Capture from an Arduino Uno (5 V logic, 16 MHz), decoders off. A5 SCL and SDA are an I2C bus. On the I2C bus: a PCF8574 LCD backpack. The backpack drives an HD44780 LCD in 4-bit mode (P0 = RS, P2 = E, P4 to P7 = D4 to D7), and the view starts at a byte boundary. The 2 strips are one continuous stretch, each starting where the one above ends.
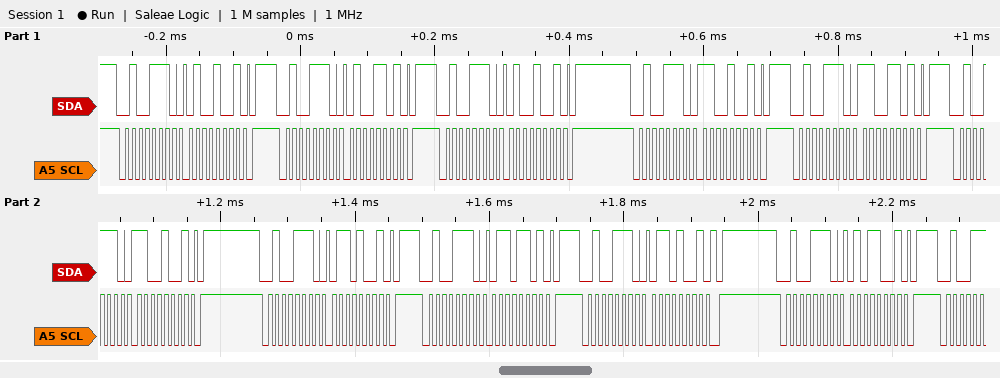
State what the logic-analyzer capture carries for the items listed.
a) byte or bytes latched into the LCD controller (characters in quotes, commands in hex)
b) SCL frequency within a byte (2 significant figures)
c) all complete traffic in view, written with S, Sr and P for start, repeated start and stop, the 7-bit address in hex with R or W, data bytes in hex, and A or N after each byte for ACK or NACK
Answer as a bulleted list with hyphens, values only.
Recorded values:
- 'L'
- 100 kHz
- S 27W A 49 A P S 27W A 4D A P S 27W A 49 A P S 27W A C9 A P S 27W A CD A P S 27W A C9 A P S 27W A 69 A P S 27W A 6D A P S 27W A 69 A P S 27W A 59 A P
